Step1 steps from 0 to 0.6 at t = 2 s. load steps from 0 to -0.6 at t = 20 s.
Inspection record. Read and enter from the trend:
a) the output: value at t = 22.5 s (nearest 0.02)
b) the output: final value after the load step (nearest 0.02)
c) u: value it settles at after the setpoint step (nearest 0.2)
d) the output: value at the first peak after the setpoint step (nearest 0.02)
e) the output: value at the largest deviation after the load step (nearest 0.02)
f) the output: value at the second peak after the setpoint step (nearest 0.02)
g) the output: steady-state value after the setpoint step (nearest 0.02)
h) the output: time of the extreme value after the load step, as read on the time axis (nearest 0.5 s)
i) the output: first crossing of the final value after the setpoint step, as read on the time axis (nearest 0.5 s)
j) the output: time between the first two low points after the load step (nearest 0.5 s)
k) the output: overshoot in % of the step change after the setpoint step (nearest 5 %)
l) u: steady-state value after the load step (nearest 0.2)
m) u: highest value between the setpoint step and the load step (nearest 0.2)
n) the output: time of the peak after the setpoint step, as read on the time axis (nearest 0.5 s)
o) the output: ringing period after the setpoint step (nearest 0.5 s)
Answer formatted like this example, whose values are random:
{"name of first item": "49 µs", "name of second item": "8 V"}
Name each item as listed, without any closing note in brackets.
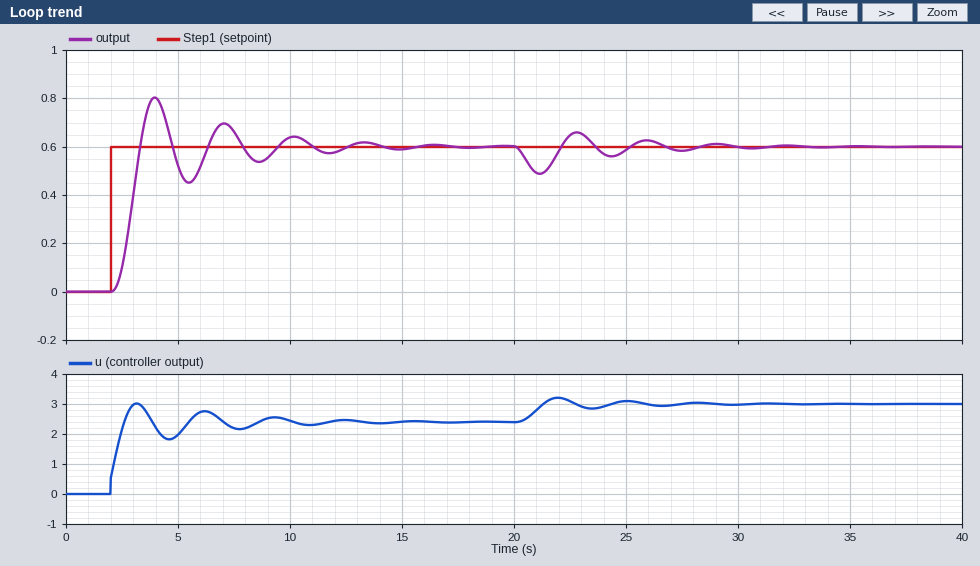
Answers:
{"the output: value at t = 22.5 s": "0.64", "the output: final value after the load step": "0.60", "u: value it settles at after the setpoint step": "2.4", "the output: value at the first peak after the setpoint step": "0.80", "the output: value at the largest deviation after the load step": "0.48", "the output: value at the second peak after the setpoint step": "0.70", "the output: steady-state value after the setpoint step": "0.60", "the output: time of the extreme value after the load step, as read on the time axis": "21.0 s", "the output: first crossing of the final value after the setpoint step, as read on the time axis": "3.5 s", "the output: time between the first two low points after the load step": "3.0 s", "the output: overshoot in % of the step change after the setpoint step": "35 %", "u: steady-state value after the load step": "3.0", "u: highest value between the setpoint step and the load step": "3.0", "the output: time of the peak after the setpoint step, as read on the time axis": "4.0 s", "the output: ringing period after the setpoint step": "3.0 s"}
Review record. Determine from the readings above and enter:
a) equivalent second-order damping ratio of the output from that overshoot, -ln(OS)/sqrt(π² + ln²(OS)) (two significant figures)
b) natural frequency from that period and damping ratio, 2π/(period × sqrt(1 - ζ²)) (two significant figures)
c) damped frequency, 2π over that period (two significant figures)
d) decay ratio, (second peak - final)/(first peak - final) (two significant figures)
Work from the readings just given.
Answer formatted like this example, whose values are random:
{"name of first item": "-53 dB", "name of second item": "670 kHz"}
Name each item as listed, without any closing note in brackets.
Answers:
{"equivalent second-order damping ratio of the output from that overshoot, -ln(OS)/sqrt(π² + ln²(OS))": "0.32", "natural frequency from that period and damping ratio, 2π/(period × sqrt(1 - ζ²))": "2.2 rad/s", "damped frequency, 2π over that period": "2.1 rad/s", "decay ratio, (second peak - final)/(first peak - final)": "0.50"}
